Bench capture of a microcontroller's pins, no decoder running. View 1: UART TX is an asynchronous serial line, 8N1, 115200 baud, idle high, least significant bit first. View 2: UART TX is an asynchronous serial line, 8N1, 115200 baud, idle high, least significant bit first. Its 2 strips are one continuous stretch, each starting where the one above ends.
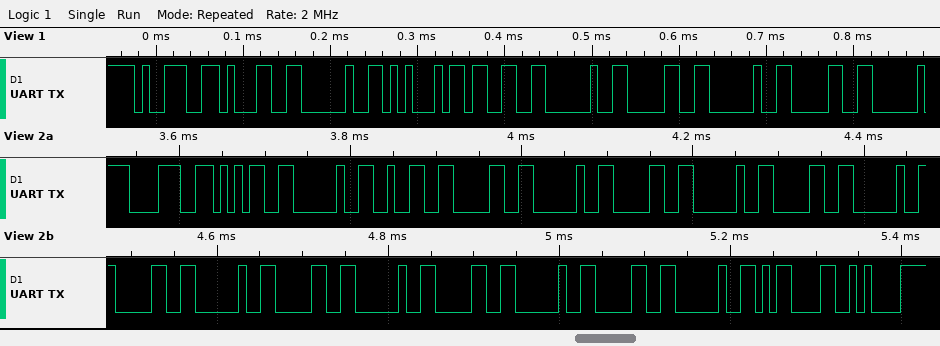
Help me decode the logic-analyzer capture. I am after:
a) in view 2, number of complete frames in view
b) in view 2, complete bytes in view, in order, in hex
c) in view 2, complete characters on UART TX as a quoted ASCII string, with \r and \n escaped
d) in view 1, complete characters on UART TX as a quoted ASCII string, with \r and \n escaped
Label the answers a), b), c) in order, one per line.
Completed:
a) 20
b) 0x38 0x35 0x20 0x32 0x30 0x20 0x30 0x20 0x30 0x20 0x30 0x20 0x30 0x20 0x30 0x20 0x30 0x20 0x0D 0x0A
c) "85 20 0 0 0 0 0 0 \r\n"
d) "91 E3 0 0"
